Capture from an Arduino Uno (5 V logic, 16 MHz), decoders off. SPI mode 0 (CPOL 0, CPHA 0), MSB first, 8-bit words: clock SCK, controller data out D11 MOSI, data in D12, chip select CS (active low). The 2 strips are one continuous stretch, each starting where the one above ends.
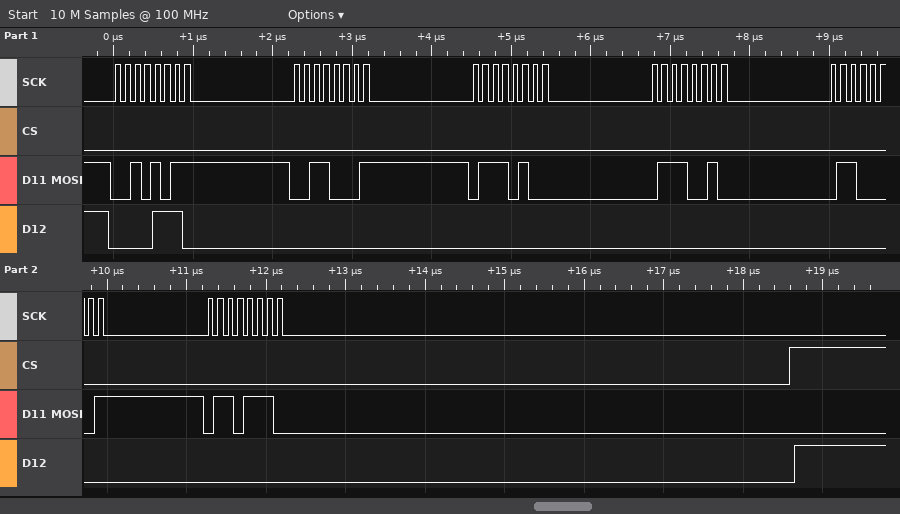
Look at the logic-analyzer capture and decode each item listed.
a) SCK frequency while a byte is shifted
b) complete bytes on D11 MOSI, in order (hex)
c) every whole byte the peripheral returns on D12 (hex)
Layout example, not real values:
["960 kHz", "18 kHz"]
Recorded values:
["8 MHz", "2B 31 74 72 61 6E", "0E 00 00 00 00 00"]
